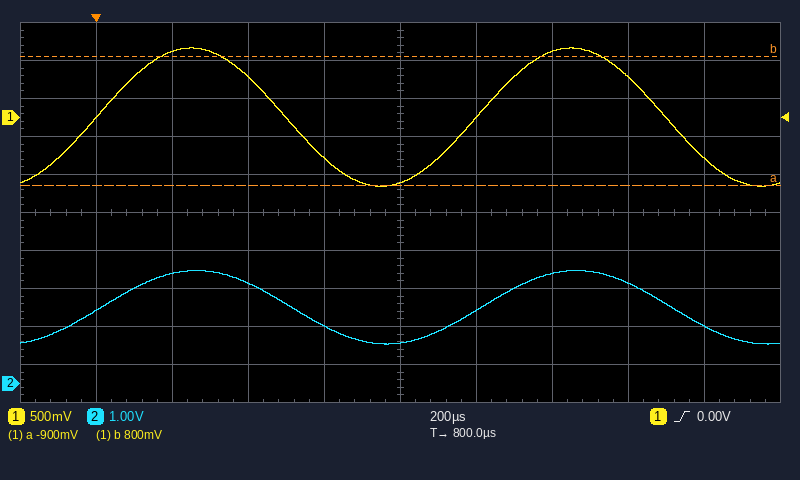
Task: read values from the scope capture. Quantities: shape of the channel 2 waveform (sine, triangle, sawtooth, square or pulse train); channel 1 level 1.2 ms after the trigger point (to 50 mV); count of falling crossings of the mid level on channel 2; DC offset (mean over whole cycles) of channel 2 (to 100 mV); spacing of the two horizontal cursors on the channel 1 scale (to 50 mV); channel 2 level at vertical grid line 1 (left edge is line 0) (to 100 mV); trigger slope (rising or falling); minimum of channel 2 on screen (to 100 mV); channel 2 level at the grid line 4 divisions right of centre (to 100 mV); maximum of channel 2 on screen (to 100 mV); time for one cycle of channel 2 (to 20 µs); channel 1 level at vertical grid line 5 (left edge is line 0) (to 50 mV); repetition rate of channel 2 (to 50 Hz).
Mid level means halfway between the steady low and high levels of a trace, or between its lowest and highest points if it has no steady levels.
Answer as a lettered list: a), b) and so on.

a) sine
b) 850 mV
c) 2
d) 2.0 V
e) 1.70 V
f) 1.9 V
g) rising
h) 1.0 V
i) 1.5 V
j) 3.0 V
k) 1.00 ms
l) -850 mV
m) 1.00 kHz
